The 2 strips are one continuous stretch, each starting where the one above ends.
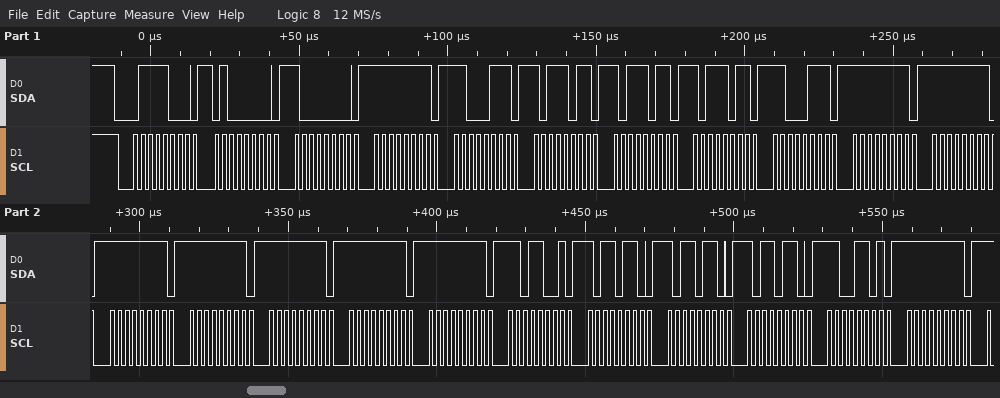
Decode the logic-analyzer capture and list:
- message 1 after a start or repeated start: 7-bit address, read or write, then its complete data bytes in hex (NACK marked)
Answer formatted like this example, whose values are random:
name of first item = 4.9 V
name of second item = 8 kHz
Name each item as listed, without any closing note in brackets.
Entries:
message 1 after a start or repeated start: 7-bit address, read or write, then its complete data bytes in hex = 0x3C write: 40 80 FF C7 BB BB BB C7 FF FF FF FF FF FF FF D9 B6 B6 B6 CD FF
